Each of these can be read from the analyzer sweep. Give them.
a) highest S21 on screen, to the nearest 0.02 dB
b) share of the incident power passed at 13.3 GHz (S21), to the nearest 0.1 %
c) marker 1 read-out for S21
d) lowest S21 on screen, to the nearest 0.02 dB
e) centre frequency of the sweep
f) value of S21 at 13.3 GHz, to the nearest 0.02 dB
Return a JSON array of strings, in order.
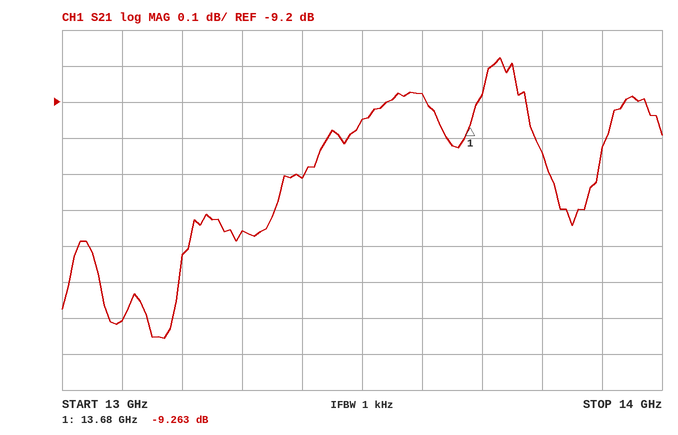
["-9.08 dB", "11.1 %", "-9.263 dB", "-9.86 dB", "13.5 GHz", "-9.56 dB"]
